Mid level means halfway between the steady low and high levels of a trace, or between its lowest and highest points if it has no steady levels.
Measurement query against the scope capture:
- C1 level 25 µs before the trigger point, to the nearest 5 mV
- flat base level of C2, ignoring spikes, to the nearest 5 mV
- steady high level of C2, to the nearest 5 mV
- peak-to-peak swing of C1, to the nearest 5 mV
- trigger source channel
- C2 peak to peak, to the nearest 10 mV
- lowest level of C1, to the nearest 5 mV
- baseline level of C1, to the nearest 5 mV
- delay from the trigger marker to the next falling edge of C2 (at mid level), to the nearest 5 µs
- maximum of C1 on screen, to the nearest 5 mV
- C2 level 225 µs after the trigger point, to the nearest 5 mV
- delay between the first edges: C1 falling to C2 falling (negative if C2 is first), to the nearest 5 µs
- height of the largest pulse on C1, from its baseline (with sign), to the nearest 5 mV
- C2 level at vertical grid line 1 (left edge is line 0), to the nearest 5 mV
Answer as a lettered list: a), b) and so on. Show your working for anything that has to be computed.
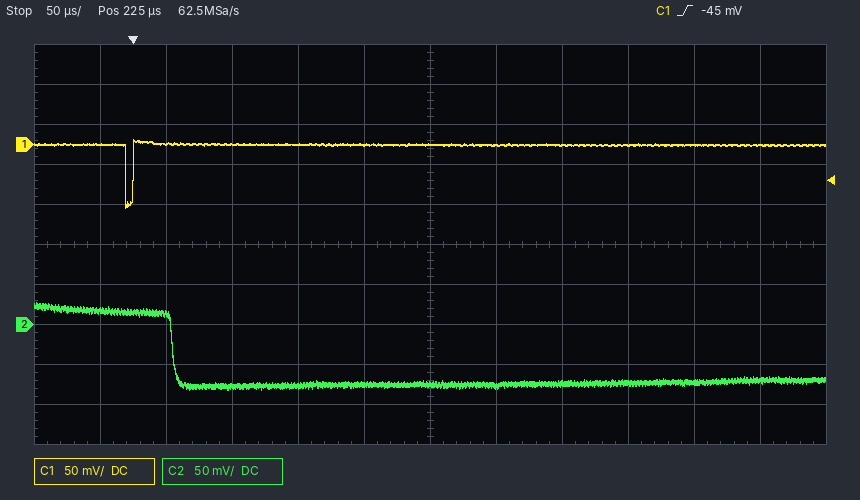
a) 0 mV
b) -75 mV
c) 15 mV
d) 5 mV − (-80 mV) = 85 mV
e) C1
f) 110 mV
g) -80 mV
h) 0 mV
i) 30 µs
j) 5 mV
k) -75 mV
l) +35 µs
m) -80 mV − (0 mV) = -80 mV
n) 15 mV
